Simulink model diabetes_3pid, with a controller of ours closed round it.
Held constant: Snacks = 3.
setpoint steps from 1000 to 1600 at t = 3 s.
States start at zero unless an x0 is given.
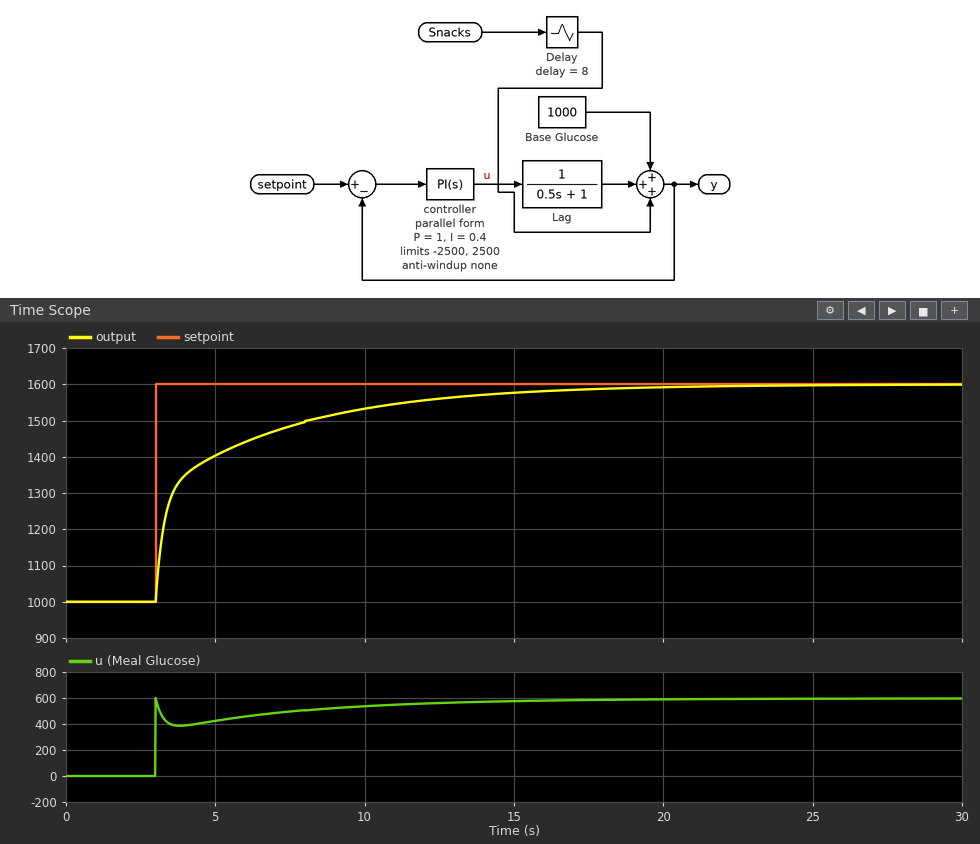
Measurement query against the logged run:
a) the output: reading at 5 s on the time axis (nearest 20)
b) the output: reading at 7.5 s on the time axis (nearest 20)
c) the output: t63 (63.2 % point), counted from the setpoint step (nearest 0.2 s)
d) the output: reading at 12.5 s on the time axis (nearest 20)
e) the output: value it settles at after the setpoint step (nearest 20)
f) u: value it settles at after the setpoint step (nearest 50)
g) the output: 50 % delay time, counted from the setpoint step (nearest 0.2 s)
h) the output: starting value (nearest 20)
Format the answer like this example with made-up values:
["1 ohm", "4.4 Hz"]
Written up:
["1400", "1480", "1.4 s", "1560", "1600", "600", "0.6 s", "1000"]
